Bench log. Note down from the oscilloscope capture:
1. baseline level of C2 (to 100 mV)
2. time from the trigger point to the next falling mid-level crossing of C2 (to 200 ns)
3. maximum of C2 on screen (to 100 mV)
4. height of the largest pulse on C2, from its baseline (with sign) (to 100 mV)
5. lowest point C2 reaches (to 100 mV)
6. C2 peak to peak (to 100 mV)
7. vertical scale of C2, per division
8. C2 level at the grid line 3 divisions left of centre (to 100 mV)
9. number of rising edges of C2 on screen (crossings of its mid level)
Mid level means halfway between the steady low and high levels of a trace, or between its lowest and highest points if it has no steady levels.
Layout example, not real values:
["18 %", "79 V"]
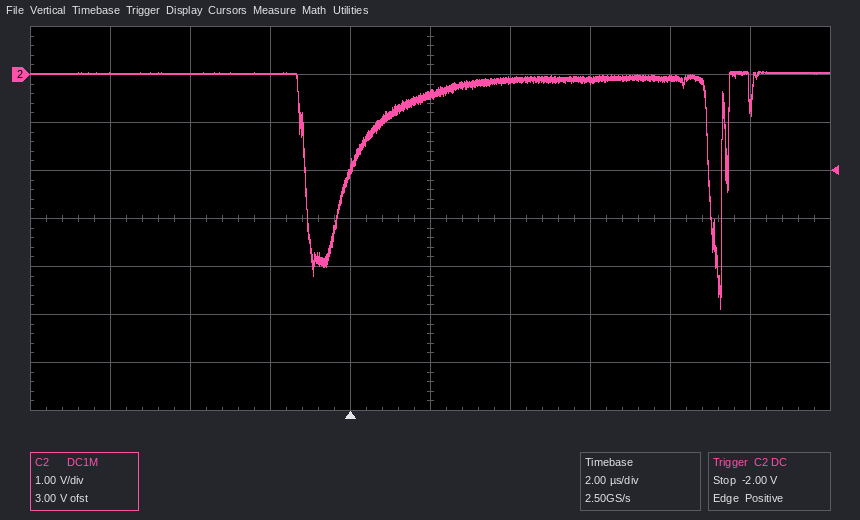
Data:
["0.0 V", "9.0 µs", "100 mV", "-4.9 V", "-4.9 V", "5.0 V", "1 V", "0.0 V", "2"]
